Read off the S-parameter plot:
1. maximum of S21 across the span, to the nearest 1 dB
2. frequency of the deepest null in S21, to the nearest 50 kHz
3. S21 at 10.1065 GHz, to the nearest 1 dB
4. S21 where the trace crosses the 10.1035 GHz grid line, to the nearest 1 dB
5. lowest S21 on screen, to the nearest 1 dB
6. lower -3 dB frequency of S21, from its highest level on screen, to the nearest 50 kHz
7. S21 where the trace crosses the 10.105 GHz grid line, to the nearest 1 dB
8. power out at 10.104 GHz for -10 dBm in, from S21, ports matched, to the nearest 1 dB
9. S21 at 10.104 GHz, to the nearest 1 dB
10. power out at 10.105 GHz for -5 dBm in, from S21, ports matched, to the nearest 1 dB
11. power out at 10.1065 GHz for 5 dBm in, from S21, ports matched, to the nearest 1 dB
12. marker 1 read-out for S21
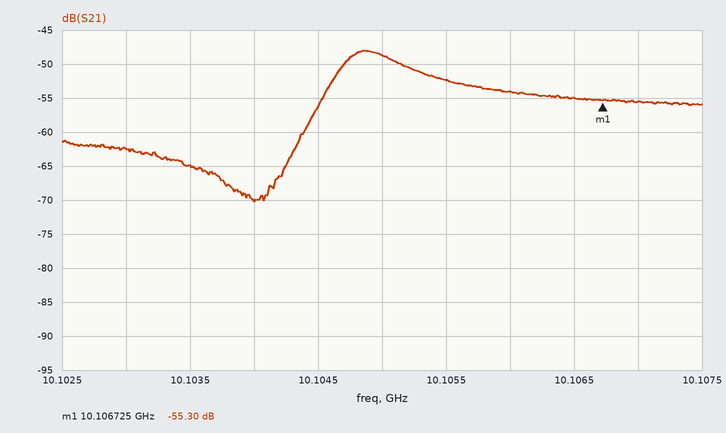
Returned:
-48 dB
10.10400 GHz
-55 dB
-65 dB
-70 dB
10.10465 GHz
-49 dB
-80 dBm
-70 dB
-54 dBm
-50 dBm
-55.30 dB
